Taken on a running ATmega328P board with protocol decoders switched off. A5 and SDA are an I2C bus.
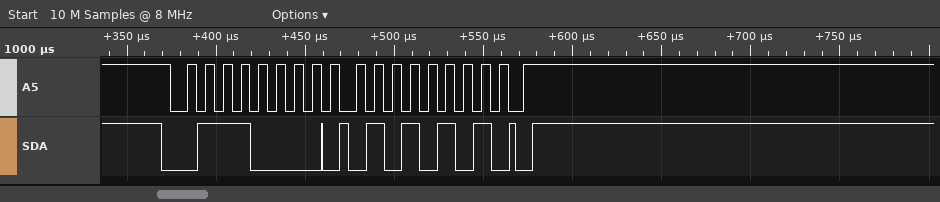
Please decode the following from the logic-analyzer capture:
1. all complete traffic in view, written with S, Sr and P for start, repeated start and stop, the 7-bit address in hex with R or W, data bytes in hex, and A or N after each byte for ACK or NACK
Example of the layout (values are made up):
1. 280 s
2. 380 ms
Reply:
1. S 38W A 55 A P
